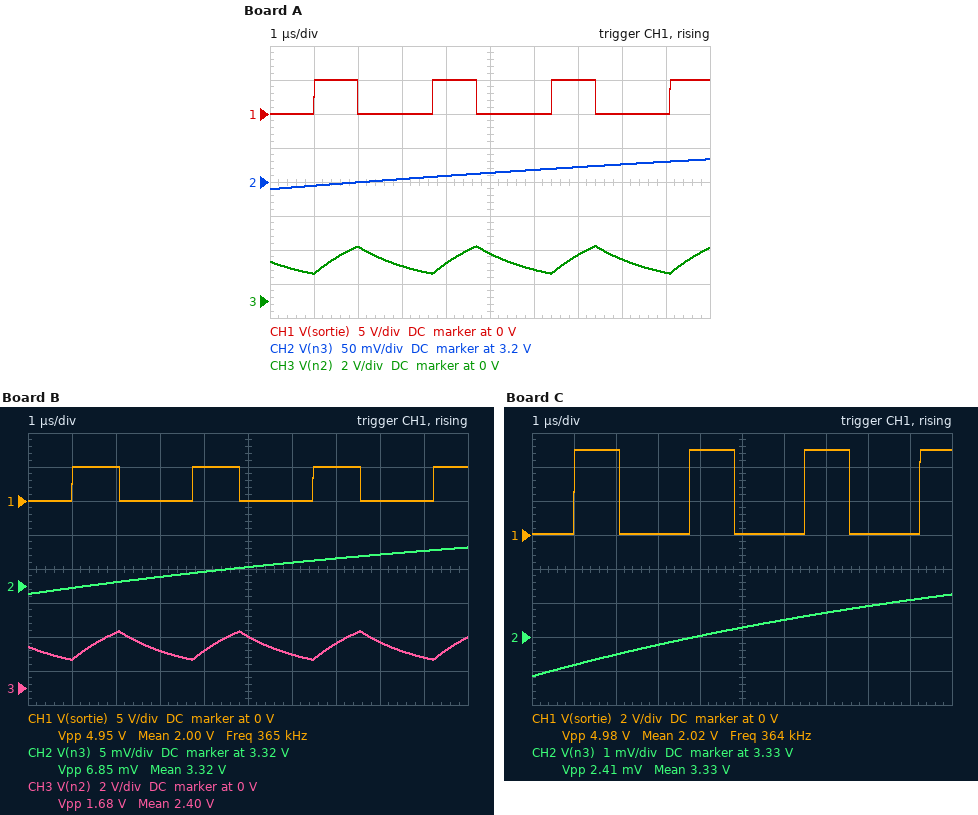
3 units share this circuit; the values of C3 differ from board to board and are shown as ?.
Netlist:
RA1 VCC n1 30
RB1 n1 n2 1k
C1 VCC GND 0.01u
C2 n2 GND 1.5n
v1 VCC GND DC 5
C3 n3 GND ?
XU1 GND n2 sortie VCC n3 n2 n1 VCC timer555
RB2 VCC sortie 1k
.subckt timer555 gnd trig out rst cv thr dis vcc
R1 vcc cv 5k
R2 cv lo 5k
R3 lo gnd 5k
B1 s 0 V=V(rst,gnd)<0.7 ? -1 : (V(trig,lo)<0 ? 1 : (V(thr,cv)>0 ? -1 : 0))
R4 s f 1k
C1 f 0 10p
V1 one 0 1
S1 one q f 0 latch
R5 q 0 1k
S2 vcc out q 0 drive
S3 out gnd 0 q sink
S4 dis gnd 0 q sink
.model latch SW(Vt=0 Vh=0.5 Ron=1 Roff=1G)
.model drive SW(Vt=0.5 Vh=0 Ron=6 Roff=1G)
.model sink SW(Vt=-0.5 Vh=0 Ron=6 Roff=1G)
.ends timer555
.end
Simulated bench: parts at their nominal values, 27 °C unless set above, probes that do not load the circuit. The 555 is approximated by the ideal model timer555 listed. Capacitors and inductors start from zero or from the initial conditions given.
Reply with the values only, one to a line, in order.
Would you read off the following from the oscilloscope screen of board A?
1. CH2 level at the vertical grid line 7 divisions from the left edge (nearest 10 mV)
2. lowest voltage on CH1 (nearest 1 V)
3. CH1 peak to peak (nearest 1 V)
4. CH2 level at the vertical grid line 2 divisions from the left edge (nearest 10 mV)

3.22 V
0 V
5 V
3.20 V
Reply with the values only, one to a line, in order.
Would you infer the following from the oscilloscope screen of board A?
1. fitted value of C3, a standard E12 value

8.2 nF
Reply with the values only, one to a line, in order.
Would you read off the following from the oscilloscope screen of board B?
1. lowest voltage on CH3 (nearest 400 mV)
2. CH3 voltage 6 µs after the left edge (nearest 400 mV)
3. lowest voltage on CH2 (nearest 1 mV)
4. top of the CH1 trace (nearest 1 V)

1.6 V
2.0 V
3.319 V
5 V
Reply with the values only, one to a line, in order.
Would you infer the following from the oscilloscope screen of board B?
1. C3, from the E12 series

4.7 nF
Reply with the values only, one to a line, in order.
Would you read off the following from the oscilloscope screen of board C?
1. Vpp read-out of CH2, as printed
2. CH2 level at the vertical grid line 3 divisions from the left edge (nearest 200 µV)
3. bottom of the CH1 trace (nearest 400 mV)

2.41 mV
3.3298 V
0 V
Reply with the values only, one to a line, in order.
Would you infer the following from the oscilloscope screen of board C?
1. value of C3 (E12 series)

3.9 nF
